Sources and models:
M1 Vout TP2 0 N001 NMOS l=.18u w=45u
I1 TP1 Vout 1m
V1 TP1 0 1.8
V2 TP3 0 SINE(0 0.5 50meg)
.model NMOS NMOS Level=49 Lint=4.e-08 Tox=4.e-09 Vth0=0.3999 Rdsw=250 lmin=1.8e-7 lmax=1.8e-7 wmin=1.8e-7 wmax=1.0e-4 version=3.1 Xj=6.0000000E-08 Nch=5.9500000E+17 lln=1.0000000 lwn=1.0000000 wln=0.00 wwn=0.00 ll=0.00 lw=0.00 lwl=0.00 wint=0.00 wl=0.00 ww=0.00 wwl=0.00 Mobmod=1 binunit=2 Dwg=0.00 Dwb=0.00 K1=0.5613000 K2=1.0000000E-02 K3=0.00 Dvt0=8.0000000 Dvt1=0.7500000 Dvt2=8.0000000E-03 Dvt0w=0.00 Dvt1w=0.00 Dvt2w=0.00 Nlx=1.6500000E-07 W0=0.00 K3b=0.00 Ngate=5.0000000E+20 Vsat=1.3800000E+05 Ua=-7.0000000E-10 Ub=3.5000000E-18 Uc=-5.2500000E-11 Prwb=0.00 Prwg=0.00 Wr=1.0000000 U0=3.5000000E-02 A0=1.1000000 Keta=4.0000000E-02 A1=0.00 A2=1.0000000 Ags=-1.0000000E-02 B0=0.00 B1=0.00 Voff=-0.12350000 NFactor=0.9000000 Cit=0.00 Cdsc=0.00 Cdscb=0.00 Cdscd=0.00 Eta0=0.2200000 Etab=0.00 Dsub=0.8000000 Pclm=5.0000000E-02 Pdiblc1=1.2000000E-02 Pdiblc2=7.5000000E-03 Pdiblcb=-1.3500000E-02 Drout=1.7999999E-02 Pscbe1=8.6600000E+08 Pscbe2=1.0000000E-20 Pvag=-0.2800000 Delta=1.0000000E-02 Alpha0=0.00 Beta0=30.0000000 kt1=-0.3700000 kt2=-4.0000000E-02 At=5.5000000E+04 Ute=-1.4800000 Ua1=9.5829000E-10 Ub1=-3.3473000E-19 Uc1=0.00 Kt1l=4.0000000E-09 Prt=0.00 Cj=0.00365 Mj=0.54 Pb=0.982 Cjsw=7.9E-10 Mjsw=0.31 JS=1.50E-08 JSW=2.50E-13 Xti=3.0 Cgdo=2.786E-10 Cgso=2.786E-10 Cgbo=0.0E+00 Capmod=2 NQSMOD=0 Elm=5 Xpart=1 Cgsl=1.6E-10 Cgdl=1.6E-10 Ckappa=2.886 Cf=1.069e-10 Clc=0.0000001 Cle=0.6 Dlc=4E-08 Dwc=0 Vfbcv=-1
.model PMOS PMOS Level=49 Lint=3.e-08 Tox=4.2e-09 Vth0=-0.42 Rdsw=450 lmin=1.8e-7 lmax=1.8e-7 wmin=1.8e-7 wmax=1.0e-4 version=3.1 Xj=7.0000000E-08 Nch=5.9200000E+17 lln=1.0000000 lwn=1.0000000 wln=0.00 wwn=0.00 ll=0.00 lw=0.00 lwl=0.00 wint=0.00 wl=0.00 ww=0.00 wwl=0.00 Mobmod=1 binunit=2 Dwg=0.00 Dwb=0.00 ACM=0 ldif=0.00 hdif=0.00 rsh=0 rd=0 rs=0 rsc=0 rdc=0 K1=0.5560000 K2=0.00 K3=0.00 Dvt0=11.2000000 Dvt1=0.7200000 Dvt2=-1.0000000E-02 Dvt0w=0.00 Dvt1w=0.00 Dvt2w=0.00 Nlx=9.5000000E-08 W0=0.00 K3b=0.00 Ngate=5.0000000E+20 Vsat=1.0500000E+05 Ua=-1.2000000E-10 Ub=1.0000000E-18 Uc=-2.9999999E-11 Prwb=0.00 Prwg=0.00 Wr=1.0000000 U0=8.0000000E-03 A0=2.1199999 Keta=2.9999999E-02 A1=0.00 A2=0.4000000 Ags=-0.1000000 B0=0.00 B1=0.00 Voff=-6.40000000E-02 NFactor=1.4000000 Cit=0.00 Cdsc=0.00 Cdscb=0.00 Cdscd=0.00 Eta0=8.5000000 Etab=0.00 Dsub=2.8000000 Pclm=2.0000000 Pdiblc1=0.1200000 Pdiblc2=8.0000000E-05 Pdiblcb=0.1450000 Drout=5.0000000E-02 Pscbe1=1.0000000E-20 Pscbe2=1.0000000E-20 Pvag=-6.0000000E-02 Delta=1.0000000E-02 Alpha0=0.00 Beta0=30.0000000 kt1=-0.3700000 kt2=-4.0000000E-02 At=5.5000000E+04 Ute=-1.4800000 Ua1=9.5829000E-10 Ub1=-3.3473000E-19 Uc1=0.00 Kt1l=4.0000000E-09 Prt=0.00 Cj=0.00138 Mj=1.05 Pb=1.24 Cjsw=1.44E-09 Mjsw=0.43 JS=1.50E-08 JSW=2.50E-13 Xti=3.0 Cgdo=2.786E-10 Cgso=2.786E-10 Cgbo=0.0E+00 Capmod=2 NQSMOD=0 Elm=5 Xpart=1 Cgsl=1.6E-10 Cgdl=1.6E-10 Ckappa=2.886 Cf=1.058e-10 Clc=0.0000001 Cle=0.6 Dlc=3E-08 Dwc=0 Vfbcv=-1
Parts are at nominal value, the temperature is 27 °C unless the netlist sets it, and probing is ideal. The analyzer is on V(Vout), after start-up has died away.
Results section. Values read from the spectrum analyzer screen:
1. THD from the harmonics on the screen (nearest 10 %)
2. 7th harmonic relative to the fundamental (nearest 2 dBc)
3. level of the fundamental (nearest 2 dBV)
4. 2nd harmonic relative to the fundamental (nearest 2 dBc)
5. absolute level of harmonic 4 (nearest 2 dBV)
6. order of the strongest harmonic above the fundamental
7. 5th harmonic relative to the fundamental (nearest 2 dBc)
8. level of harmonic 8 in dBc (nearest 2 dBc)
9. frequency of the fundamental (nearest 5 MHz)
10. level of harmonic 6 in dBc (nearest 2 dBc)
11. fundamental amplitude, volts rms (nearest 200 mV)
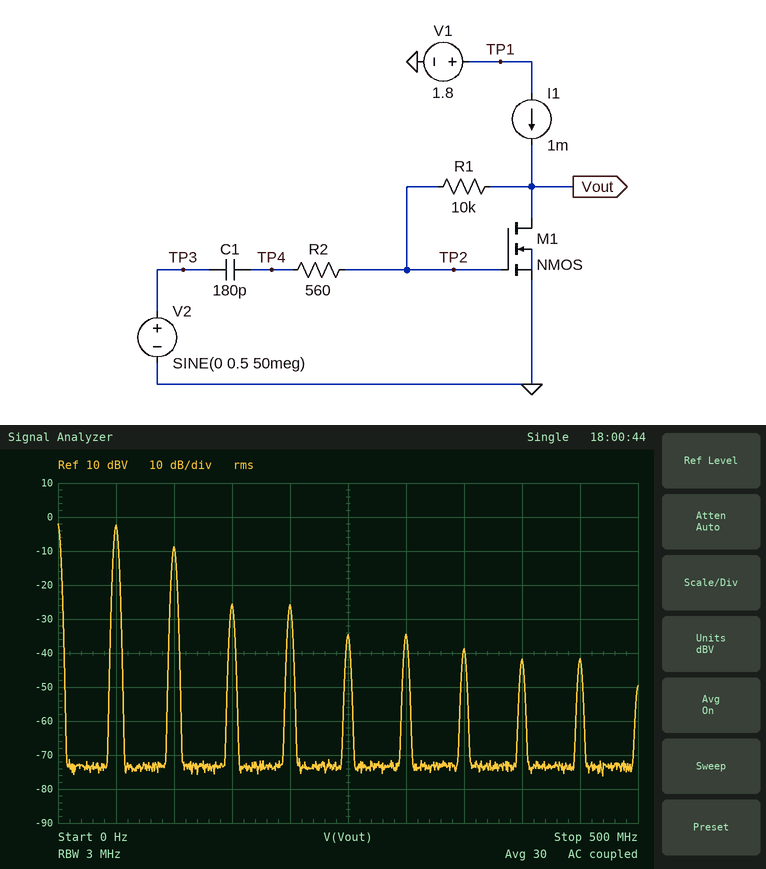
50 %
-36 dBc
-2 dBV
-6 dBc
-26 dBV
2
-32 dBc
-40 dBc
50 MHz
-32 dBc
800 mV
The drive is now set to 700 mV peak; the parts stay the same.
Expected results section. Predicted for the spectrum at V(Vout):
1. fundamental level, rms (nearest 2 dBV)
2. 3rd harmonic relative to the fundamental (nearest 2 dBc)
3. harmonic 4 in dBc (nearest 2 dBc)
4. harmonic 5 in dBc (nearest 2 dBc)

0 dBV
-18 dBc
-24 dBc
-26 dBc
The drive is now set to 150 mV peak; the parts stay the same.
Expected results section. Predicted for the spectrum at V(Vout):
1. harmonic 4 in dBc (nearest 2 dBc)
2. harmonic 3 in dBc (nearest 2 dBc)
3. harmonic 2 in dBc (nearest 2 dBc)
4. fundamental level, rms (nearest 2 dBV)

-48 dBc
-24 dBc
-14 dBc
-8 dBV
